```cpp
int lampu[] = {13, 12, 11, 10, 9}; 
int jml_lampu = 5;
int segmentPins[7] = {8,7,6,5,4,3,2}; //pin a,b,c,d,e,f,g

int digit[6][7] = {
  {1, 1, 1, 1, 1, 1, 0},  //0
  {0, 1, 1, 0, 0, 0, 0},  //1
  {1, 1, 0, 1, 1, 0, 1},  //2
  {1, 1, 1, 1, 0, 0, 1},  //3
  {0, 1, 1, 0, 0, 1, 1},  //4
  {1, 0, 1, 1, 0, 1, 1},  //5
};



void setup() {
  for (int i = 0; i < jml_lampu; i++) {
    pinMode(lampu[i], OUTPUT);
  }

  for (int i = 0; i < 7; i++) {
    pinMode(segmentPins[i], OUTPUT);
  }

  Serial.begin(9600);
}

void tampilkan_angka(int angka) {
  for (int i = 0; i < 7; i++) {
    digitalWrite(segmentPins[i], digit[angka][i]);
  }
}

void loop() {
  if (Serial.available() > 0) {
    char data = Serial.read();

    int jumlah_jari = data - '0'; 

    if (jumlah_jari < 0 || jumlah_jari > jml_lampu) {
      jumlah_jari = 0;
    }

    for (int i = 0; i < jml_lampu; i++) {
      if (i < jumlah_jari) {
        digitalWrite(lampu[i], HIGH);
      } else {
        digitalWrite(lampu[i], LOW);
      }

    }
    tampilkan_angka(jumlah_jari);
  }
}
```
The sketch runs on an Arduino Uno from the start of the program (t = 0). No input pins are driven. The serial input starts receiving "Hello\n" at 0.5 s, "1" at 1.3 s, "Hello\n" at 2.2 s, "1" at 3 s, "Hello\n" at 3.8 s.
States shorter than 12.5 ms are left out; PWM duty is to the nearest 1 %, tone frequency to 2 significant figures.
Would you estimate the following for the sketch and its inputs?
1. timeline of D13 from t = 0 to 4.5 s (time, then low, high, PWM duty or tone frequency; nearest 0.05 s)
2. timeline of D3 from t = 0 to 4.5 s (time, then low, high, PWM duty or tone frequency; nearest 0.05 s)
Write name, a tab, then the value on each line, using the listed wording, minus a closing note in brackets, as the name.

timeline of D13 from t = 0 to 4.5 s	0 s low; 1.3 s high; 2.2 s low; 3 s high; 3.8 s low
timeline of D3 from t = 0 to 4.5 s	0 s low; 0.5 s high; 1.3 s low; 2.2 s high; 3 s low; 3.8 s high
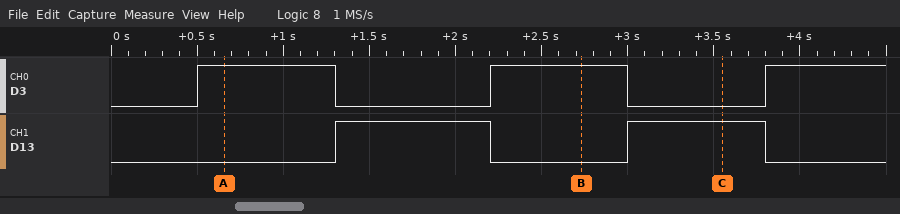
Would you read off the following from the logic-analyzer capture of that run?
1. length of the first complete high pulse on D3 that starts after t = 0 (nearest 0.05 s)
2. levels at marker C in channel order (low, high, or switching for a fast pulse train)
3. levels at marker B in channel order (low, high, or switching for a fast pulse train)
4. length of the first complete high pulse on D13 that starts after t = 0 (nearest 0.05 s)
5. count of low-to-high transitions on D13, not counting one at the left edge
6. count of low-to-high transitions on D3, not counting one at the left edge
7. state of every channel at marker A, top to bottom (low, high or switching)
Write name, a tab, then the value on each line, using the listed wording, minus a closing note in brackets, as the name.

length of the first complete high pulse on D3 that starts after t = 0	0.80 s
levels at marker C in channel order	D3 low, D13 high
levels at marker B in channel order	D3 high, D13 low
length of the first complete high pulse on D13 that starts after t = 0	0.90 s
count of low-to-high transitions on D13, not counting one at the left edge	2
count of low-to-high transitions on D3, not counting one at the left edge	3
state of every channel at marker A, top to bottom	D3 high, D13 low
